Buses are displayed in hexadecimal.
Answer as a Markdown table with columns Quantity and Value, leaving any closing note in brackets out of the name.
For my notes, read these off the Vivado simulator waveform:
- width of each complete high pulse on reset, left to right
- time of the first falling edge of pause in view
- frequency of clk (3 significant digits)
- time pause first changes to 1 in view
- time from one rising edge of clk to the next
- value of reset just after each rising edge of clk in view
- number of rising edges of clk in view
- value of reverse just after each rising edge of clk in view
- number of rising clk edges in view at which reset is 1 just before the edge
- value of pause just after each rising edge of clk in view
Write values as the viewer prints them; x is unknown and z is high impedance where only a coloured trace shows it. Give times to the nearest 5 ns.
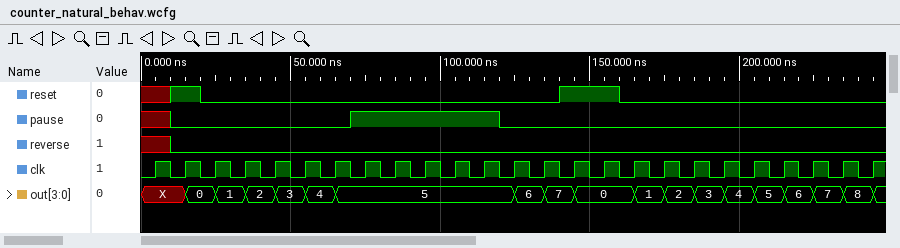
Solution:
| Quantity | Value |
|---|---|
| width of each complete high pulse on reset, left to right | 20 ns |
| time of the first falling edge of pause in view | 120 ns |
| frequency of clk | 100 MHz |
| time pause first changes to 1 in view | 70 ns |
| time from one rising edge of clk to the next | 10 ns |
| value of reset just after each rising edge of clk in view | x 1 0 0 0 0 0 0 0 0 0 0 0 0 1 1 0 0 0 0 0 0 0 0 0 |
| number of rising edges of clk in view | 25 |
| value of reverse just after each rising edge of clk in view | x 0 0 0 0 0 0 0 0 0 0 0 0 0 0 0 0 0 0 0 0 0 0 0 0 |
| number of rising clk edges in view at which reset is 1 just before the edge | 3 |
| value of pause just after each rising edge of clk in view | x 0 0 0 0 0 0 1 1 1 1 1 0 0 0 0 0 0 0 0 0 0 0 0 0 |
